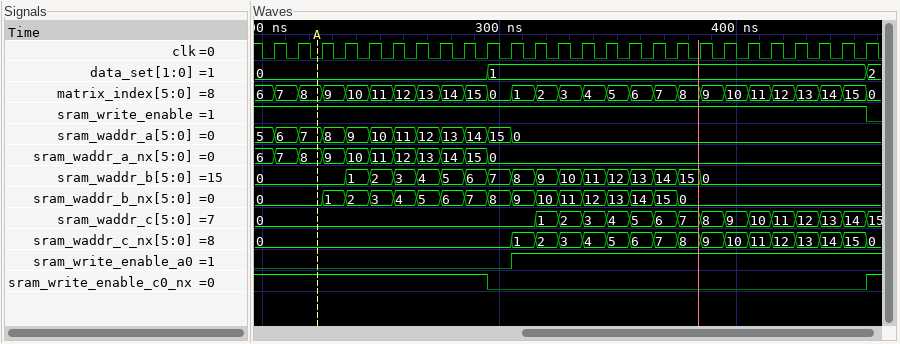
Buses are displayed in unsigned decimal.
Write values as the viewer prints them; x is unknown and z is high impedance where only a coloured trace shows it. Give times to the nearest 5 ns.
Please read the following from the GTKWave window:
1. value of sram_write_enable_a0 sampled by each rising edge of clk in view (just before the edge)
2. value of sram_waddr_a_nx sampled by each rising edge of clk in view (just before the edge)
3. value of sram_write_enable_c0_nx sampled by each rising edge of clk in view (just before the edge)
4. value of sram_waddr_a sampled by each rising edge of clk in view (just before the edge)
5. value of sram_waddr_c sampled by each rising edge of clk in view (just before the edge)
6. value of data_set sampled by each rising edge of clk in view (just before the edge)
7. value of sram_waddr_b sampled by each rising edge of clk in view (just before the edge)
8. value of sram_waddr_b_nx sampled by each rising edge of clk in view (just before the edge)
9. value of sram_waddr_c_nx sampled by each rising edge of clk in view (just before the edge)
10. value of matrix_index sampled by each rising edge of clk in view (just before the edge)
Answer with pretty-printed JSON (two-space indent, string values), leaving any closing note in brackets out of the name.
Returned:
{
  "value of sram_write_enable_a0 sampled by each rising edge of clk in view": "0 0 0 0 0 0 0 0 0 0 0 1 1 1 1 1 1 1 1 1 1 1 1 1 1 1",
  "value of sram_waddr_a_nx sampled by each rising edge of clk in view": "6, 7, 8, 9, 10, 11, 12, 13, 14, 15, 0, 0, 0, 0, 0, 0, 0, 0, 0, 0, 0, 0, 0, 0, 0, 0",
  "value of sram_write_enable_c0_nx sampled by each rising edge of clk in view": "1 1 1 1 1 1 1 1 1 1 0 0 0 0 0 0 0 0 0 0 0 0 0 0 0 0",
  "value of sram_waddr_a sampled by each rising edge of clk in view": "5, 6, 7, 8, 9, 10, 11, 12, 13, 14, 15, 0, 0, 0, 0, 0, 0, 0, 0, 0, 0, 0, 0, 0, 0, 0",
  "value of sram_waddr_c sampled by each rising edge of clk in view": "0, 0, 0, 0, 0, 0, 0, 0, 0, 0, 0, 0, 1, 2, 3, 4, 5, 6, 7, 8, 9, 10, 11, 12, 13, 14",
  "value of data_set sampled by each rising edge of clk in view": "0, 0, 0, 0, 0, 0, 0, 0, 0, 0, 1, 1, 1, 1, 1, 1, 1, 1, 1, 1, 1, 1, 1, 1, 1, 1",
  "value of sram_waddr_b sampled by each rising edge of clk in view": "0, 0, 0, 0, 1, 2, 3, 4, 5, 6, 7, 8, 9, 10, 11, 12, 13, 14, 15, 0, 0, 0, 0, 0, 0, 0",
  "value of sram_waddr_b_nx sampled by each rising edge of clk in view": "0, 0, 0, 1, 2, 3, 4, 5, 6, 7, 8, 9, 10, 11, 12, 13, 14, 15, 0, 0, 0, 0, 0, 0, 0, 0",
  "value of sram_waddr_c_nx sampled by each rising edge of clk in view": "0, 0, 0, 0, 0, 0, 0, 0, 0, 0, 0, 1, 2, 3, 4, 5, 6, 7, 8, 9, 10, 11, 12, 13, 14, 15",
  "value of matrix_index sampled by each rising edge of clk in view": "6, 7, 8, 9, 10, 11, 12, 13, 14, 15, 0, 1, 2, 3, 4, 5, 6, 7, 8, 9, 10, 11, 12, 13, 14, 15"
}
